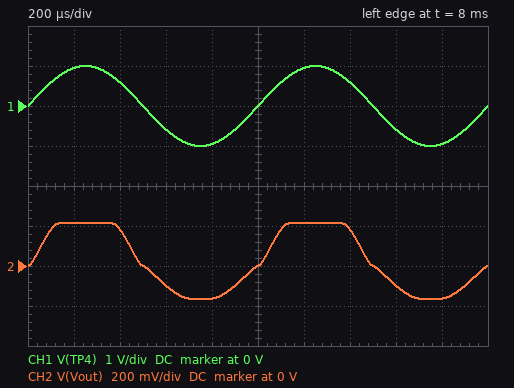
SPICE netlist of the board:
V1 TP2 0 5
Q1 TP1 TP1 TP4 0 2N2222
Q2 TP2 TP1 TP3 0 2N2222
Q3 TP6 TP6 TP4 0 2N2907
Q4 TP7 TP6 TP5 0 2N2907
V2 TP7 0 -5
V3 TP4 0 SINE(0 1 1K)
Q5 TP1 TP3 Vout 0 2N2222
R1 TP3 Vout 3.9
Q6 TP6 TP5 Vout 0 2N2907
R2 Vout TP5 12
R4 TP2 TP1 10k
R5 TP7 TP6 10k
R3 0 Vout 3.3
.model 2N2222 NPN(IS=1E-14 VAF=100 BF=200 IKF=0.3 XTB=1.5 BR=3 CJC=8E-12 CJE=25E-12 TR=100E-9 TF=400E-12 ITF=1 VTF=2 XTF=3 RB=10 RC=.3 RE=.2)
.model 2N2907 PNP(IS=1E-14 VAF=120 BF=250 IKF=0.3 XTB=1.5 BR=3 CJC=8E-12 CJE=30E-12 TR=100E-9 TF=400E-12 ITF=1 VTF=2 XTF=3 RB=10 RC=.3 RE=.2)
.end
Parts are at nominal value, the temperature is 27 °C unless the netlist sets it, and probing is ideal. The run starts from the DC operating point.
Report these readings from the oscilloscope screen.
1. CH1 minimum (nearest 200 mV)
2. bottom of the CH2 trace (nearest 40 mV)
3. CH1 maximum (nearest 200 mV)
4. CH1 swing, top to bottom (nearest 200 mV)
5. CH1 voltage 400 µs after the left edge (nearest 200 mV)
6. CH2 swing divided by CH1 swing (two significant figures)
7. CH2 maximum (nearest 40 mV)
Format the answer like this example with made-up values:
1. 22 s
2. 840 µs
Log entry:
1. -1.0 V
2. -160 mV
3. 1.0 V
4. 2.0 V
5. 600 mV
6. 0.19
7. 200 mV
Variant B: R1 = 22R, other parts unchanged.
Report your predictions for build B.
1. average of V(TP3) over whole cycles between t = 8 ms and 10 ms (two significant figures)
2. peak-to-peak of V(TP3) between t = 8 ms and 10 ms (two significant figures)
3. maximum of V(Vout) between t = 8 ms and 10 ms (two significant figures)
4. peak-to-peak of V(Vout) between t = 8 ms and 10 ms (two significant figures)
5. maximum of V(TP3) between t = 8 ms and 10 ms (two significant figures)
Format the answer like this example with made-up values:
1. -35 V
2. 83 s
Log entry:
1. 190 mV
2. 870 mV
3. 93 mV
4. 260 mV
5. 710 mV
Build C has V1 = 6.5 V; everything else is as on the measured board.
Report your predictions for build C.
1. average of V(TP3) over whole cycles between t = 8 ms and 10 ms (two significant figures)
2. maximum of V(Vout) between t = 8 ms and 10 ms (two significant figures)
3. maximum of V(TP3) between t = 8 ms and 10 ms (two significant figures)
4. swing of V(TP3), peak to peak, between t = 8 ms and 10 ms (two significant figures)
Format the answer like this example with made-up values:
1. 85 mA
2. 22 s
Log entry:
1. 160 mV
2. 280 mV
3. 610 mV
4. 780 mV
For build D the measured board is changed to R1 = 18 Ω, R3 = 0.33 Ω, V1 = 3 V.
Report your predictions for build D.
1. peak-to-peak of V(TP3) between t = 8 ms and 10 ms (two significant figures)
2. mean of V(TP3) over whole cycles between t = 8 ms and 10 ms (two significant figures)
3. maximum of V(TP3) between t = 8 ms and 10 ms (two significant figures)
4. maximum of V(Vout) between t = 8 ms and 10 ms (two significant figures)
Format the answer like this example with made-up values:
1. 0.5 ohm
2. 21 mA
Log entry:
1. 560 mV
2. 190 mV
3. 550 mV
4. 9.8 mV
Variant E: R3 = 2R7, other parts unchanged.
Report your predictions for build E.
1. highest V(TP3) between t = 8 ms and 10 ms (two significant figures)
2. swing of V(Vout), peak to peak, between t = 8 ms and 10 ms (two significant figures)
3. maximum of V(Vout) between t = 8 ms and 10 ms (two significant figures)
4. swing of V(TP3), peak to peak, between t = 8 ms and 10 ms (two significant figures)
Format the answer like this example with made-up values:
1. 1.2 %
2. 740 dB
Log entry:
1. 430 mV
2. 310 mV
3. 180 mV
4. 570 mV
